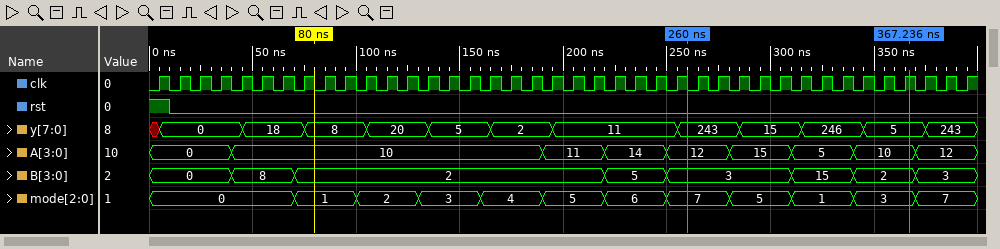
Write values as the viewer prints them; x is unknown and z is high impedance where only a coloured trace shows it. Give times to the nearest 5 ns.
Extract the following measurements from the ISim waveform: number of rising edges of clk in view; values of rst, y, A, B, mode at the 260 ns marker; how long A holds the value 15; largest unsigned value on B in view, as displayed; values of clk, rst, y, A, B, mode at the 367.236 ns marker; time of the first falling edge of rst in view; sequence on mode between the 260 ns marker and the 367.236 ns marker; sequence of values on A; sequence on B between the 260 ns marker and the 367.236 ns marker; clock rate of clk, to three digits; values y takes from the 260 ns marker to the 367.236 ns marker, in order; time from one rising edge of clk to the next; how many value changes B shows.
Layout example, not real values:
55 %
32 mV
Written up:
40
rst=0, y=243, A=12, B=3, mode=7
30 ns
15
clk=1, rst=0, y=5, A=10, B=2, mode=3
10 ns
7, 5, 1, 3
0, 10, 11, 14, 12, 15, 5, 10, 12
3, 15, 2
100 MHz
243, 15, 246, 5
10 ns
7
